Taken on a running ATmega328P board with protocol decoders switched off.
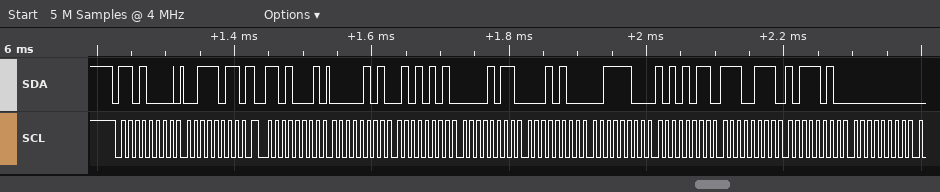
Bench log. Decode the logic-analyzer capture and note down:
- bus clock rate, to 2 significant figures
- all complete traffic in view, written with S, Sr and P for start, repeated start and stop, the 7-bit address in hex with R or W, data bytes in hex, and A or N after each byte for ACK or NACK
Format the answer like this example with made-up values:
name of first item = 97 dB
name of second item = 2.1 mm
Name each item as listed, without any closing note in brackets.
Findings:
bus clock rate, to 2 significant figures = 100 kHz
all complete traffic in view, written with S, Sr and P for start, repeated start and stop, the 7-bit address in hex with R or W, data bytes in hex, and A or N after each byte for ACK or NACK = S 68W A 3B A Sr 68R A 05 A 55 A 0B A 14 A 3C A AB A E7 A BA A 00 A
